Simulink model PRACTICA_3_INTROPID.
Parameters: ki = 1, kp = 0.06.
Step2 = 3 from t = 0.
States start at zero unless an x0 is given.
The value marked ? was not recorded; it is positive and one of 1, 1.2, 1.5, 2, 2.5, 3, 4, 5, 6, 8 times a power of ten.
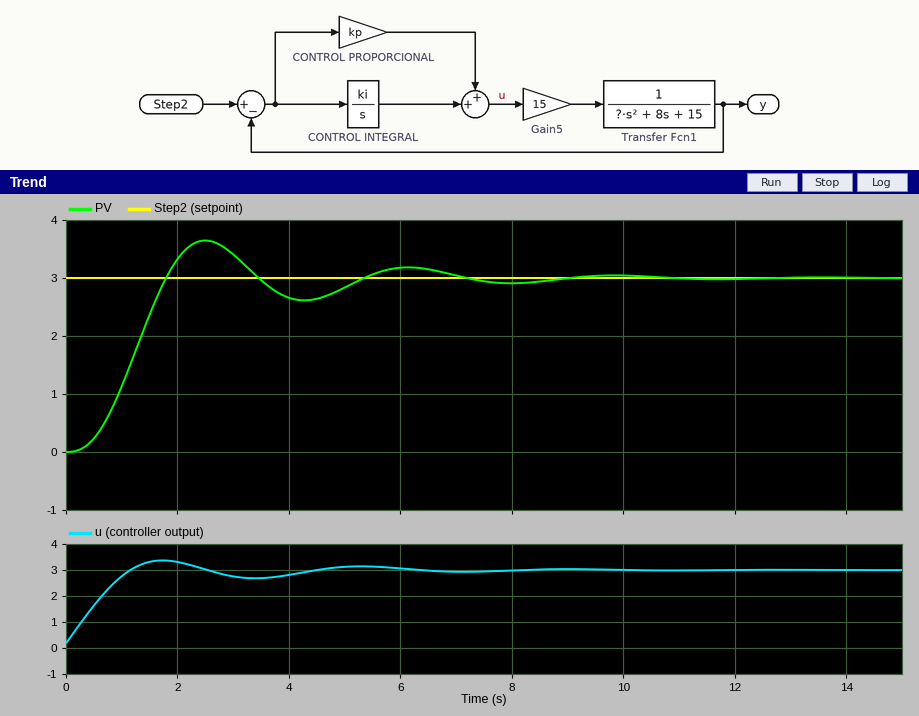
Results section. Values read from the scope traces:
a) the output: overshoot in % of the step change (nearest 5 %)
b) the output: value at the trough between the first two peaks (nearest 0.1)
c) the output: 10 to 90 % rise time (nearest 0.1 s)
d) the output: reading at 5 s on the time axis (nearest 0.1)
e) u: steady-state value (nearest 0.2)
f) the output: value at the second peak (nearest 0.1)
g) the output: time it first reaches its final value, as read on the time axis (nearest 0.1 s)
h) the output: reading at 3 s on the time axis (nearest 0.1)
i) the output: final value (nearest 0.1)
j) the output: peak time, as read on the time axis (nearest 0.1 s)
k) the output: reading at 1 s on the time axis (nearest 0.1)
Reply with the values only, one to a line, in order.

20 %
2.6
1.1 s
2.8
3.0
3.2
1.8 s
3.4
3.0
2.5 s
1.1
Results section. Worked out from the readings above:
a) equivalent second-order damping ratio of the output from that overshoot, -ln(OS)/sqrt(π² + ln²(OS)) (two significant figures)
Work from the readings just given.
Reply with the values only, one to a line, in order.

0.46
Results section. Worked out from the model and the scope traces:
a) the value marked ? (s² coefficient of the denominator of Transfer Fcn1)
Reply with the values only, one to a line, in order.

4
